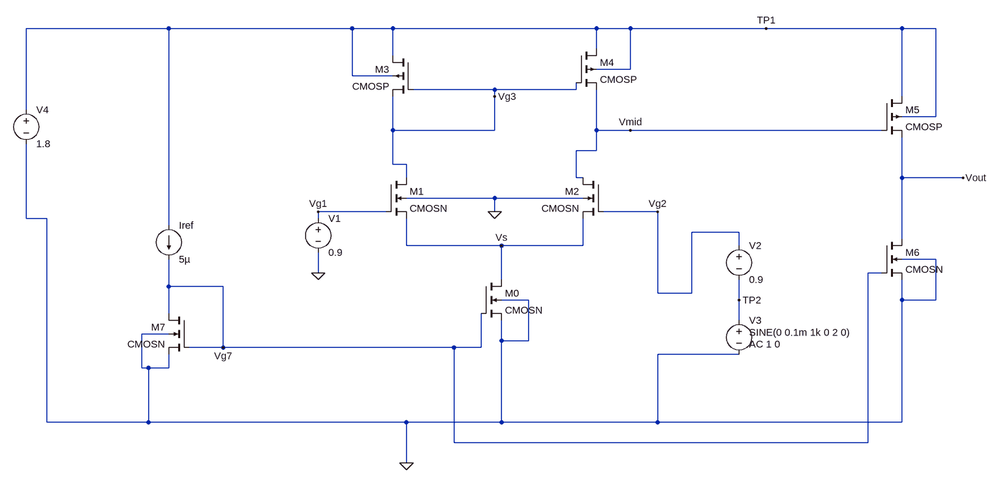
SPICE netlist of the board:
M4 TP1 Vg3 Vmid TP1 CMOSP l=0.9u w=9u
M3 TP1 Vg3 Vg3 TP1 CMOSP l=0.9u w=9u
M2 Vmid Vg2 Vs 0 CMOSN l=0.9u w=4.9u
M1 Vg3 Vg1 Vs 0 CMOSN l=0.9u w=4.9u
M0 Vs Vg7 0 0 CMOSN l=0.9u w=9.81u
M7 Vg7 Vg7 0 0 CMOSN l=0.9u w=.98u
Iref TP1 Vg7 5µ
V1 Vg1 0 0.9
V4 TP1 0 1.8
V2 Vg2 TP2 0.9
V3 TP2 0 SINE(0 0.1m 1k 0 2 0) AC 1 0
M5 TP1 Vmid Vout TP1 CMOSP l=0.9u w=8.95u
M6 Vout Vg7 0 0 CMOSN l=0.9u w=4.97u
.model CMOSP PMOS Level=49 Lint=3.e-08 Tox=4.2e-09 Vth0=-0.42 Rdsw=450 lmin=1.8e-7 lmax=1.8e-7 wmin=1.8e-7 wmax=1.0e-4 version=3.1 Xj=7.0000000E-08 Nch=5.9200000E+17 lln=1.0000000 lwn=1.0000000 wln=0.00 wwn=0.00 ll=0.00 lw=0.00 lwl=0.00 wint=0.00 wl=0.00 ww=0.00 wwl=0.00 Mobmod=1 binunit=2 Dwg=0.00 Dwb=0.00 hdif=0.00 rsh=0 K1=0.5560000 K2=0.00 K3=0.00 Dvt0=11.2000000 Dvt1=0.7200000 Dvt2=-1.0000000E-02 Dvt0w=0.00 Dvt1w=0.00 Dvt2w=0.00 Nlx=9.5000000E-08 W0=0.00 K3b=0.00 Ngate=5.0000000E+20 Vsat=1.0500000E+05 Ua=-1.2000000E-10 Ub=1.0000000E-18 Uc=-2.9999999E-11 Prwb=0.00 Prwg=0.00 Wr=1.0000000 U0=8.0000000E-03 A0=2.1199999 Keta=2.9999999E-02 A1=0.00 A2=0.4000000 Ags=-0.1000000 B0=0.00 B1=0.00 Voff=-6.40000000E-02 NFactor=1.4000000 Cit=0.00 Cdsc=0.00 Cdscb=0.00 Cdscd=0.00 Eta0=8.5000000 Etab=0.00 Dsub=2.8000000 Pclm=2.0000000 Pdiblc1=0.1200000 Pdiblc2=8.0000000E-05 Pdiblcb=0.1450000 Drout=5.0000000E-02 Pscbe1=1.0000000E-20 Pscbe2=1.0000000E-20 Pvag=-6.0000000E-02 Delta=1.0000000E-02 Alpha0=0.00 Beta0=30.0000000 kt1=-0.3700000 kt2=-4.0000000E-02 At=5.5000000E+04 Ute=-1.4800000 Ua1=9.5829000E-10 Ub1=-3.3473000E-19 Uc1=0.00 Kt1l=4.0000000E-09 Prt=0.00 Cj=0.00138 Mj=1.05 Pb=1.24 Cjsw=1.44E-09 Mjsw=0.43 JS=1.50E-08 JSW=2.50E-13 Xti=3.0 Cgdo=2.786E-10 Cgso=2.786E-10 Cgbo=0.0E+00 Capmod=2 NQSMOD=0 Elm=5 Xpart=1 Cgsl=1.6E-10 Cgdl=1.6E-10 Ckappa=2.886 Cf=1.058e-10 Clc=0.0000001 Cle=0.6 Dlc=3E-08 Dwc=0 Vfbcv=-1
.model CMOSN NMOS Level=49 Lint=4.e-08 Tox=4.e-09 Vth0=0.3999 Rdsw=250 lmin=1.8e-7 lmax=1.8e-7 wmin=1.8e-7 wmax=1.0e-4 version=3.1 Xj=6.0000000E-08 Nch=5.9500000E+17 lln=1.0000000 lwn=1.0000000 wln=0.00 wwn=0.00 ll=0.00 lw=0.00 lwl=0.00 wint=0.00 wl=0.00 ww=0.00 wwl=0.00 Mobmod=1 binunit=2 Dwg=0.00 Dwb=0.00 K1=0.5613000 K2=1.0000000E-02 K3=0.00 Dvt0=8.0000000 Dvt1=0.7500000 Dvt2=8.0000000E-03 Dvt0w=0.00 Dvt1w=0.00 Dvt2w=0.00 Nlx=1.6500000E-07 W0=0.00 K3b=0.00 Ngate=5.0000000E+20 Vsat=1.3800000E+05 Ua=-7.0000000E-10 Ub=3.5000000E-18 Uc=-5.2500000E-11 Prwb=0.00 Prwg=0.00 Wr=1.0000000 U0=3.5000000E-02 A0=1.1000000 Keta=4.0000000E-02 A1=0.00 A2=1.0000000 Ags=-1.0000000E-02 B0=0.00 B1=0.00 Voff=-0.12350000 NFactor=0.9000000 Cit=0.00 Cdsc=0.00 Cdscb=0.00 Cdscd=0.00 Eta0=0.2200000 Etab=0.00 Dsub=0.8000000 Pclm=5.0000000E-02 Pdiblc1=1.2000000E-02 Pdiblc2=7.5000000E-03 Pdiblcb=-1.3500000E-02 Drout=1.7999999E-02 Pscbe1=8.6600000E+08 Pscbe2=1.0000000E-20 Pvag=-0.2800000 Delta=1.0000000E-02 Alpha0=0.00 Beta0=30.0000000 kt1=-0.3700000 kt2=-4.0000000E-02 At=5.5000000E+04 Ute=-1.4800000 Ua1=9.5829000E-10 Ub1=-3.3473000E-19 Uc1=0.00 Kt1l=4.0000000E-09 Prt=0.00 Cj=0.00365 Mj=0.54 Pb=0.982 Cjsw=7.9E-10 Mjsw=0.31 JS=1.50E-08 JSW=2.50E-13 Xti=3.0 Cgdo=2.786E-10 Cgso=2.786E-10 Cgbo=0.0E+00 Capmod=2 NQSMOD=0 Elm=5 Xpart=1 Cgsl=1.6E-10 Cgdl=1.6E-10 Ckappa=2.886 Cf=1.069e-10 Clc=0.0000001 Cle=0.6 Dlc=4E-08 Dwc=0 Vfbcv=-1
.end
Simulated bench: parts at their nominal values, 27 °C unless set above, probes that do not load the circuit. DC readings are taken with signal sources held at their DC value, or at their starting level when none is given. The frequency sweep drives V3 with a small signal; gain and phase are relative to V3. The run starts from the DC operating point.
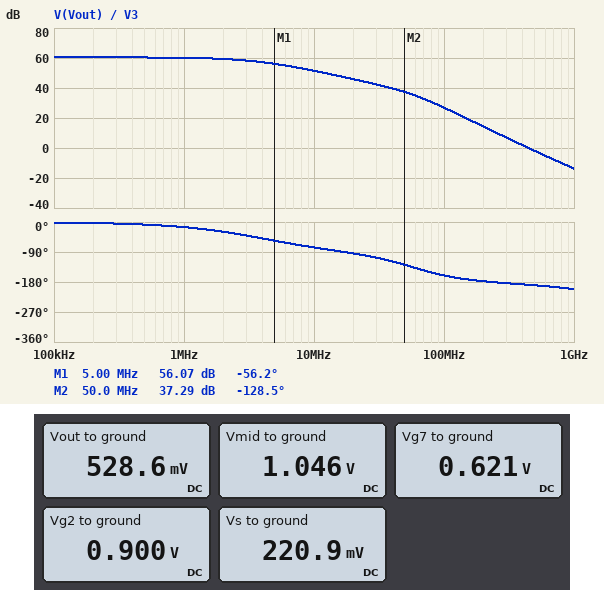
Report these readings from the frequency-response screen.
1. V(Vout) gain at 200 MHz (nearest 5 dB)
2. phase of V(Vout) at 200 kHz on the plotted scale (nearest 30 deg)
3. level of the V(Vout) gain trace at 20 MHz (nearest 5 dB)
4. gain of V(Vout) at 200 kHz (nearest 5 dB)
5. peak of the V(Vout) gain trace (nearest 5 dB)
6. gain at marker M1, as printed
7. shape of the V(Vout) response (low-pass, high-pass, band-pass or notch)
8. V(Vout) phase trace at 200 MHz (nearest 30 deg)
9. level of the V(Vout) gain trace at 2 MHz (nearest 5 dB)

15 dB
0 deg
45 dB
60 dB
60 dB
56.07 dB
low-pass
-180 deg
60 dB
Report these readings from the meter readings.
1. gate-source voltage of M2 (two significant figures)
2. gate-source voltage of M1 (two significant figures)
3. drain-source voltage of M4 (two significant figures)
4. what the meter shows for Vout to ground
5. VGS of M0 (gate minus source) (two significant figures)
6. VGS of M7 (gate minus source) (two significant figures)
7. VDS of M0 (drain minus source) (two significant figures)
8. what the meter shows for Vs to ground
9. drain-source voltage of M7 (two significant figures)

680 mV
680 mV
750 mV
528.6 mV
620 mV
620 mV
220 mV
220.9 mV
620 mV
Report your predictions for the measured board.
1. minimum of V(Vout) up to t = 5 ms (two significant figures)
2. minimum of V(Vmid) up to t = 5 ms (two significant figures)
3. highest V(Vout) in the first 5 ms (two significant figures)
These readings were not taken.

420 mV
1.0 V
630 mV
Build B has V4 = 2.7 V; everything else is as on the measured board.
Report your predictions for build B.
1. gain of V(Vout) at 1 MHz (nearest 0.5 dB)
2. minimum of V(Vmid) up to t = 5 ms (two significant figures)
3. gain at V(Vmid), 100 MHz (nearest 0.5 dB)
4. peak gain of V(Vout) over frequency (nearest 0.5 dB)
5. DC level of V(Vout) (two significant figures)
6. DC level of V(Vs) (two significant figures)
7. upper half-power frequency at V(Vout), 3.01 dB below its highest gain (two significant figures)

61.0 dB
1.9 V
10.5 dB
61.5 dB
1.0 V
230 mV
3.7 MHz
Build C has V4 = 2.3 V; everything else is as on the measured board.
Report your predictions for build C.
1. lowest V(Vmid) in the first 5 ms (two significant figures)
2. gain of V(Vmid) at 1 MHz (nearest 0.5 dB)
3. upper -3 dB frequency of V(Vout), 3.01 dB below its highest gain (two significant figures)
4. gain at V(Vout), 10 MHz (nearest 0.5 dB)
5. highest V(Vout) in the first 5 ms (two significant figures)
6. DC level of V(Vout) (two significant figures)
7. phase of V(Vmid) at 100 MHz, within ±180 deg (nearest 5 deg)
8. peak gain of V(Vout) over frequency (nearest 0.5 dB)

1.5 V
32.0 dB
3.7 MHz
52.0 dB
910 mV
800 mV
85 deg
61.0 dB
